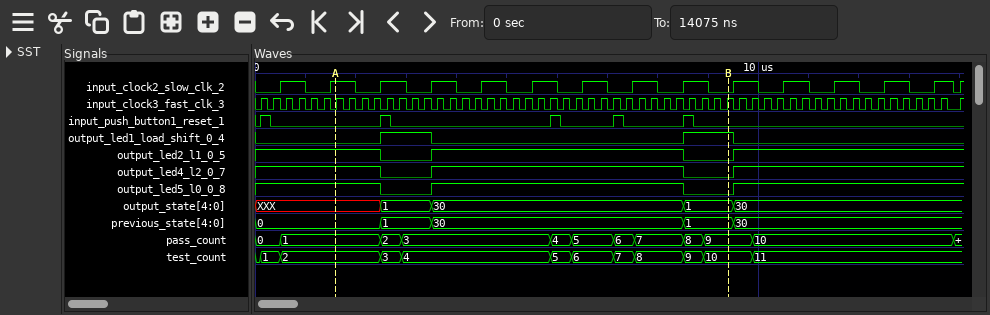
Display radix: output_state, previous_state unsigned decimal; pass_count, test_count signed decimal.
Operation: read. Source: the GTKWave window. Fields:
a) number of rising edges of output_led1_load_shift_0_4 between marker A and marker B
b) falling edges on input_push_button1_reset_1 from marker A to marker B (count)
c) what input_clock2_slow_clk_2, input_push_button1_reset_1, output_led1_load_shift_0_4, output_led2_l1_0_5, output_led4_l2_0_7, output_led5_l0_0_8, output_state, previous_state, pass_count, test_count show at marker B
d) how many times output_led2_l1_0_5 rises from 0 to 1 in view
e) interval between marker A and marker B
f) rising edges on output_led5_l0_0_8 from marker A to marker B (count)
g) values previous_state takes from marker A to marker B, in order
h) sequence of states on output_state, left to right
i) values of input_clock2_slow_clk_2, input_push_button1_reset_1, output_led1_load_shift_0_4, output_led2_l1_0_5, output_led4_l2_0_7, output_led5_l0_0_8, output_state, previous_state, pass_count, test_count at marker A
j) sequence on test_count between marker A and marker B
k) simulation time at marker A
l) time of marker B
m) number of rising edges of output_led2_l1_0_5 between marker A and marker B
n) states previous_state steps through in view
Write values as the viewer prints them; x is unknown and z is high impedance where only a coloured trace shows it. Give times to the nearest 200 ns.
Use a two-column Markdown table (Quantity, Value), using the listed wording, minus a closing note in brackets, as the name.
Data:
| Quantity | Value |
|---|---|
| number of rising edges of output_led1_load_shift_0_4 between marker A and marker B | 2 |
| falling edges on input_push_button1_reset_1 from marker A to marker B | 4 |
| what input_clock2_slow_clk_2, input_push_button1_reset_1, output_led1_load_shift_0_4, output_led2_l1_0_5, output_led4_l2_0_7, output_led5_l0_0_8, output_state, previous_state, pass_count, test_count show at marker B | input_clock2_slow_clk_2=0, input_push_button1_reset_1=0, output_led1_load_shift_0_4=1, output_led2_l1_0_5=0, output_led4_l2_0_7=0, output_led5_l0_0_8=0, output_state=1, previous_state=1, pass_count=9, test_count=10 |
| how many times output_led2_l1_0_5 rises from 0 to 1 in view | 2 |
| interval between marker A and marker B | 7800 ns |
| rising edges on output_led5_l0_0_8 from marker A to marker B | 1 |
| values previous_state takes from marker A to marker B, in order | 0, 1, 30, 1 |
| sequence of states on output_state, left to right | XXX, 1, 30, 1, 30 |
| values of input_clock2_slow_clk_2, input_push_button1_reset_1, output_led1_load_shift_0_4, output_led2_l1_0_5, output_led4_l2_0_7, output_led5_l0_0_8, output_state, previous_state, pass_count, test_count at marker A | input_clock2_slow_clk_2=1, input_push_button1_reset_1=0, output_led1_load_shift_0_4=0, output_led2_l1_0_5=1, output_led4_l2_0_7=1, output_led5_l0_0_8=1, output_state=XXX, previous_state=0, pass_count=1, test_count=2 |
| sequence on test_count between marker A and marker B | 2, 3, 4, 5, 6, 7, 8, 9, 10 |
| simulation time at marker A | 1600 ns |
| time of marker B | 9400 ns |
| number of rising edges of output_led2_l1_0_5 between marker A and marker B | 1 |
| states previous_state steps through in view | 0, 1, 30, 1, 30 |
